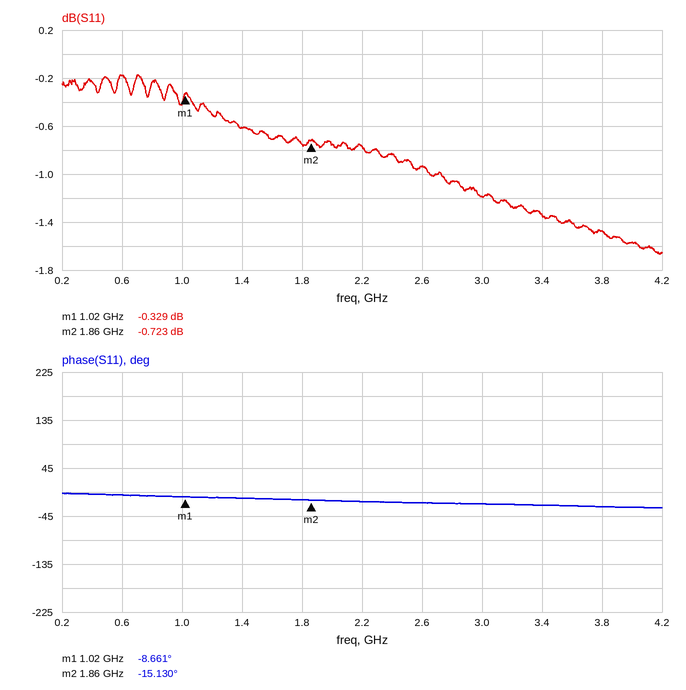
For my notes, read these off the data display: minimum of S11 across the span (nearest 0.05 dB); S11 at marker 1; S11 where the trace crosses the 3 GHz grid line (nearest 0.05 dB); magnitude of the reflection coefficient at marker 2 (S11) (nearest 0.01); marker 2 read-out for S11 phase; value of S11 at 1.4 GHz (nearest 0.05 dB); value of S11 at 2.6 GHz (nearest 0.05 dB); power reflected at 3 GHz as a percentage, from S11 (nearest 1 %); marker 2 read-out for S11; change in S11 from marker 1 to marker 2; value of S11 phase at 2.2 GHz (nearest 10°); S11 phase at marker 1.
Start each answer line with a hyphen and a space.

- -1.65 dB
- -0.329 dB
- -1.20 dB
- 0.92
- -15.130°
- -0.60 dB
- -0.95 dB
- 76 %
- -0.723 dB
- -0.394 dB
- -20°
- -8.661°
